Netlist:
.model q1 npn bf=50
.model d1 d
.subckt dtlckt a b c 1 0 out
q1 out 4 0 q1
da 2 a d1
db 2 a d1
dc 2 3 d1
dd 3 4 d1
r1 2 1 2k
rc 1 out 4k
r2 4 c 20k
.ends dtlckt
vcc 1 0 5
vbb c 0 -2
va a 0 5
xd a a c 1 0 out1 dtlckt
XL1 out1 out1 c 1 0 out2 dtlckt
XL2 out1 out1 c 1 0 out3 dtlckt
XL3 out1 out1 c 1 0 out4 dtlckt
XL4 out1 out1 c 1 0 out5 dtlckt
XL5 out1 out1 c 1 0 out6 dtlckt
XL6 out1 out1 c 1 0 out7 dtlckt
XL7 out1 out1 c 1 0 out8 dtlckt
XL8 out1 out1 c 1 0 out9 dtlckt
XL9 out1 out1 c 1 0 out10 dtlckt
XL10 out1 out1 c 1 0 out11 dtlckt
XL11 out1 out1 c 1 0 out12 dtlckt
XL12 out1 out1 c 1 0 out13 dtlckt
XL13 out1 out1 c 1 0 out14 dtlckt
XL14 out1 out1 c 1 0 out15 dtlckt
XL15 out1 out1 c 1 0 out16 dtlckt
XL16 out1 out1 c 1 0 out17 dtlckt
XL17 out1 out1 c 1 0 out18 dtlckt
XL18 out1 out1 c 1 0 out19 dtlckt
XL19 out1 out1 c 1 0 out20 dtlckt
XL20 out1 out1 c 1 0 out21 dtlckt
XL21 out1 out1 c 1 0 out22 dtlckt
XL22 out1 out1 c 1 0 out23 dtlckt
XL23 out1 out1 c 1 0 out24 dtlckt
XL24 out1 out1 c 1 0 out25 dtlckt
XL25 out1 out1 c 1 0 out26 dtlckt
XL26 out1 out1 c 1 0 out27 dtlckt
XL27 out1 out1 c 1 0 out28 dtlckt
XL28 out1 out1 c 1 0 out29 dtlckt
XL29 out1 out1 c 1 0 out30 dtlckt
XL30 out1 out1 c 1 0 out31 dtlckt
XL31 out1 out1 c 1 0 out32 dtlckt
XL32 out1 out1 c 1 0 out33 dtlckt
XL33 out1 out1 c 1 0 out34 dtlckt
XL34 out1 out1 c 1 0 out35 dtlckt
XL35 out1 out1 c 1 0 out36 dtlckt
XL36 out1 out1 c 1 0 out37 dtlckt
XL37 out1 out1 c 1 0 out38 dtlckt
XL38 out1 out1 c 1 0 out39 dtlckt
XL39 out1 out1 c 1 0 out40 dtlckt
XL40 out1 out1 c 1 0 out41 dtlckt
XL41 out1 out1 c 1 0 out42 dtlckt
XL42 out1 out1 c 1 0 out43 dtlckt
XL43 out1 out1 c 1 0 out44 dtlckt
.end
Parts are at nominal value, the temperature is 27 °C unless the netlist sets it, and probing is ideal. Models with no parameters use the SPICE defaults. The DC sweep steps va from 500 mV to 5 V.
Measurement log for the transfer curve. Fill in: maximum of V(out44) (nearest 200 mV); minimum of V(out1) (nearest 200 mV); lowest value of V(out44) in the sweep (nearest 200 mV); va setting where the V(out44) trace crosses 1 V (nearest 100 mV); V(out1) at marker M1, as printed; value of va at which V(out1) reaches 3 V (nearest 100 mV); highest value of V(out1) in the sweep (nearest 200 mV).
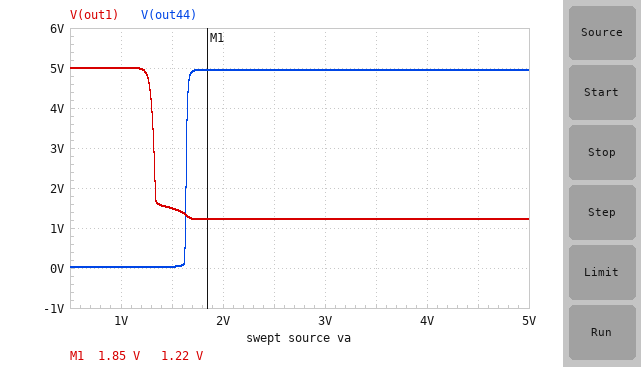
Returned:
5.0 V
1.2 V
0 V
1.6 V
1.22 V
1.3 V
5.0 V
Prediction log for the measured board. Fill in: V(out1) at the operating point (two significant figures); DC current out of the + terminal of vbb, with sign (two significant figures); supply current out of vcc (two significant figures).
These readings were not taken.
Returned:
1.2 V
-5.9 mA
70 mA
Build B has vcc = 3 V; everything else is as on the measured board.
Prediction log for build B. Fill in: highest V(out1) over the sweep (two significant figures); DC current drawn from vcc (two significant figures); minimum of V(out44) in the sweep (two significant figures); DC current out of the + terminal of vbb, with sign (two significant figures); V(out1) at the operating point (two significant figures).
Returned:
3.0 V
54 mA
38 mV
-6.1 mA
1.4 V
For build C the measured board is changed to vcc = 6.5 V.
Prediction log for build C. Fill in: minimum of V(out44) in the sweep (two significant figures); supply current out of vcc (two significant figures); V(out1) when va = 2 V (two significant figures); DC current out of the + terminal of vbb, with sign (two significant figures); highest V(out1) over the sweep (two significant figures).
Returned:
27 mV
110 mA
1.0 V
-5.5 mA
6.5 V
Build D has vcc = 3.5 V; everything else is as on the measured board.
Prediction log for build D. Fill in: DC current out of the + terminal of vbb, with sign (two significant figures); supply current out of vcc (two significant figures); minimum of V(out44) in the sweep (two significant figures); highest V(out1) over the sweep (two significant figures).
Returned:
-6.1 mA
66 mA
33 mV
3.5 V
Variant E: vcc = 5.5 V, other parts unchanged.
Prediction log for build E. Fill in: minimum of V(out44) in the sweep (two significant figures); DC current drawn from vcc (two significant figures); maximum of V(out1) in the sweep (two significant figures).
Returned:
28 mV
82 mA
5.5 V
